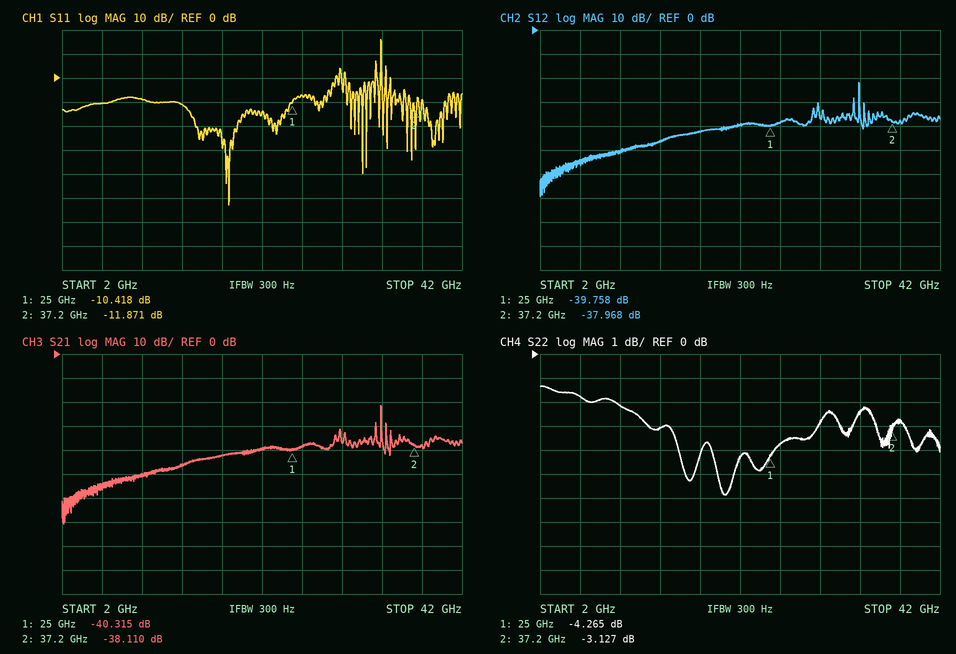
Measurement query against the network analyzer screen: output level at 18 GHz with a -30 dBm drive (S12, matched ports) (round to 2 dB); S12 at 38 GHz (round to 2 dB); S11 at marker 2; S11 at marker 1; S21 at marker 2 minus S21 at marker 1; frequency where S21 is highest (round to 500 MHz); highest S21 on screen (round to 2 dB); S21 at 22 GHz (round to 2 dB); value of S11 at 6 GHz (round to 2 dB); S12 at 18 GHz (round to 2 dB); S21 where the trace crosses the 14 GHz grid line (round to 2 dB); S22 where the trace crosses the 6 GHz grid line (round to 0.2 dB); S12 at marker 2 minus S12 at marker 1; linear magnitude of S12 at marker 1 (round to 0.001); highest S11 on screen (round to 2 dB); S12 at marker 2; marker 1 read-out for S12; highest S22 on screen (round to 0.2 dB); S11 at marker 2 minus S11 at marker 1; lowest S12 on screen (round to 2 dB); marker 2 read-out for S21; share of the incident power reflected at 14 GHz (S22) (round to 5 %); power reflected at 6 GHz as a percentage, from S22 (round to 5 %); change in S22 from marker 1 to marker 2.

-72 dBm
-38 dB
-11.871 dB
-10.418 dB
2.205 dB
34.0 GHz
-22 dB
-40 dB
-10 dB
-42 dB
-46 dB
-1.8 dB
1.790 dB
0.010
16 dB
-37.968 dB
-39.758 dB
-1.4 dB
-1.453 dB
-70 dB
-38.110 dB
50 %
65 %
1.138 dB
